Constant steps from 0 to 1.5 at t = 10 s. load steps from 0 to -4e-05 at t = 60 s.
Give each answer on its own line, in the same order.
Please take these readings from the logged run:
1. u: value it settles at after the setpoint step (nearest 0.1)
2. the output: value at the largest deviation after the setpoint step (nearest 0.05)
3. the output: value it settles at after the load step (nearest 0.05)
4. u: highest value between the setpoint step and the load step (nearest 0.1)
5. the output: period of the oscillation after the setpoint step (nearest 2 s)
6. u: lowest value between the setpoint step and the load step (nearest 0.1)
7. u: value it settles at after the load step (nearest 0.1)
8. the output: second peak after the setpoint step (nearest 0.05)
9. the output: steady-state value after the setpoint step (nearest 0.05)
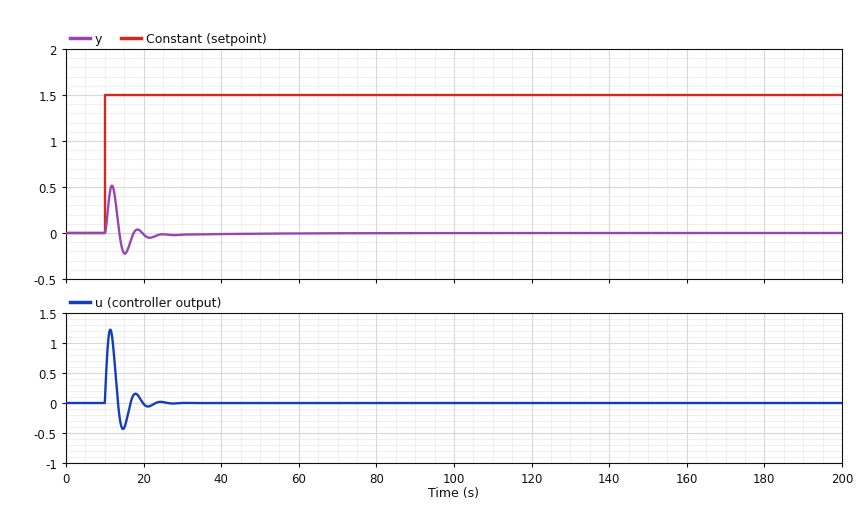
0.0
0.50
0.00
1.2
6 s
-0.4
0.0
0.05
0.00
